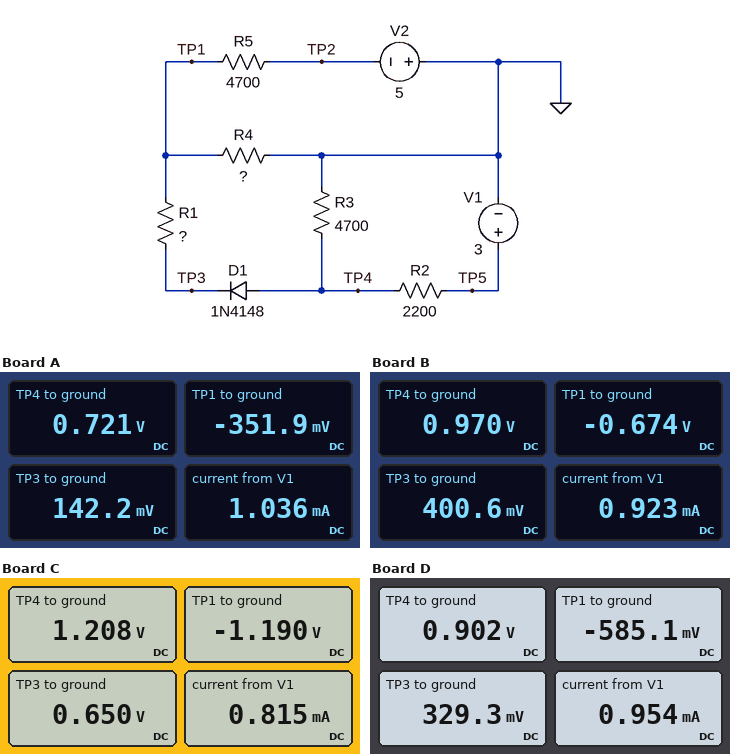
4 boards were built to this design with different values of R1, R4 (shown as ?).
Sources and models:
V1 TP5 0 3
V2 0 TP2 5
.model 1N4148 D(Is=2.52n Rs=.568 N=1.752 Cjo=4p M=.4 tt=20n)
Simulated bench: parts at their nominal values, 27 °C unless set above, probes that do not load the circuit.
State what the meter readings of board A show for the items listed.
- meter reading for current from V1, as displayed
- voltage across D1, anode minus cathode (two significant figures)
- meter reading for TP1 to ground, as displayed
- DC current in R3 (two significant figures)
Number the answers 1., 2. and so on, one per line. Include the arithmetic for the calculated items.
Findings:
1. 1.036 mA
2. 721 mV - 142.2 mV = 580 mV
3. -351.9 mV
4. (721 mV) / 4.7 kΩ = 150 µA
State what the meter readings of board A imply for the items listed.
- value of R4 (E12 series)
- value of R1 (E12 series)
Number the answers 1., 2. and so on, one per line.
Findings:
1. 3.3 kΩ
2. 560 Ω
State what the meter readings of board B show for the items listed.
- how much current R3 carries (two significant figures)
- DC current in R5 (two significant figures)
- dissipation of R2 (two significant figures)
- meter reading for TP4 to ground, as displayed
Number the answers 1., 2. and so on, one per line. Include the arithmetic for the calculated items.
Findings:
1. (970 mV) / 4.7 kΩ = 210 µA
2. (-674 mV - (-5 V)) / 4.7 kΩ = 920 µA
3. (3 V - 970 mV)^2 / 2.2 kΩ = 1.9 mW
4. 0.970 V
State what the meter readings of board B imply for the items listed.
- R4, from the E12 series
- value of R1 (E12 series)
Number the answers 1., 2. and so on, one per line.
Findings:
1. 3.3 kΩ
2. 1.5 kΩ
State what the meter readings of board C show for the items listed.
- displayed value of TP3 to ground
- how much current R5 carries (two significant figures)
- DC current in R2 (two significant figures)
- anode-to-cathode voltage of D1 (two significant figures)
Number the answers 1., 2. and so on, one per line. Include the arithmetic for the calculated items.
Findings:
1. 0.650 V
2. (-1.19 V - (-5 V)) / 4.7 kΩ = 810 µA
3. (3 V - 1.208 V) / 2.2 kΩ = 810 µA
4. 1.208 V - 650 mV = 560 mV
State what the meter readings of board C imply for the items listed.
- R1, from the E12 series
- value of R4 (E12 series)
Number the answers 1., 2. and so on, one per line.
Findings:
1. 3.3 kΩ
2. 4.7 kΩ
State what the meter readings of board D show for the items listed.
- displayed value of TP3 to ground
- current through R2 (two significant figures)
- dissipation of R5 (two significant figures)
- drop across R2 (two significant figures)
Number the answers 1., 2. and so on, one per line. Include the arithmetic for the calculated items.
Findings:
1. 329.3 mV
2. (3 V - 902 mV) / 2.2 kΩ = 950 µA
3. (-585.1 mV - (-5 V))^2 / 4.7 kΩ = 4.1 mW
4. 3 V - 902 mV = 2.1 V
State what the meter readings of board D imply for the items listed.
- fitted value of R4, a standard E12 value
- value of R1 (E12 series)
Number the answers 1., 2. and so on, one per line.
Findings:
1. 3.3 kΩ
2. 1.2 kΩ
